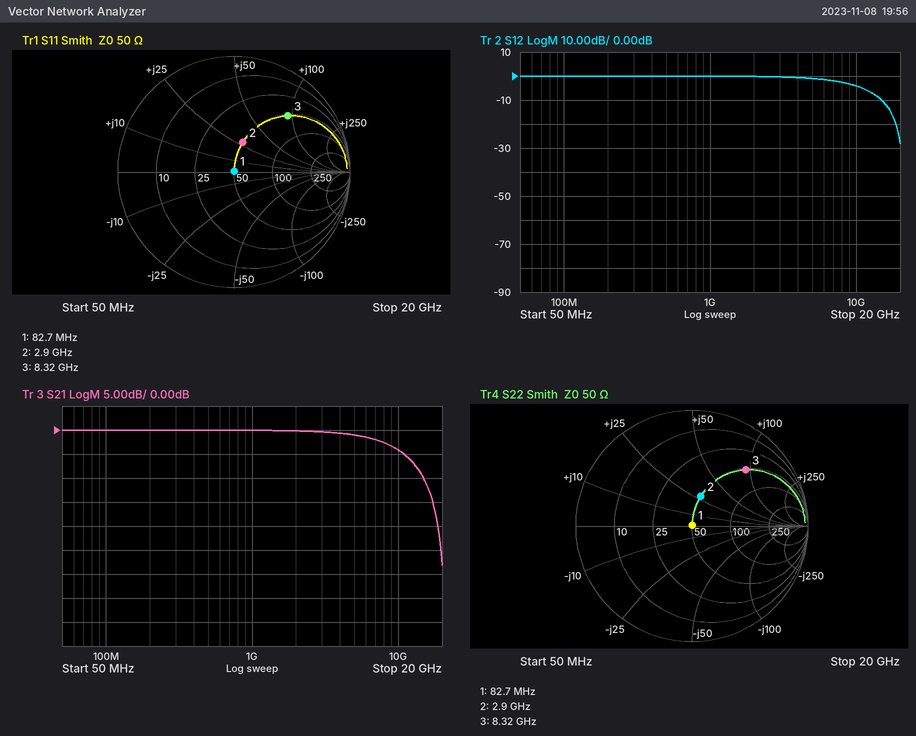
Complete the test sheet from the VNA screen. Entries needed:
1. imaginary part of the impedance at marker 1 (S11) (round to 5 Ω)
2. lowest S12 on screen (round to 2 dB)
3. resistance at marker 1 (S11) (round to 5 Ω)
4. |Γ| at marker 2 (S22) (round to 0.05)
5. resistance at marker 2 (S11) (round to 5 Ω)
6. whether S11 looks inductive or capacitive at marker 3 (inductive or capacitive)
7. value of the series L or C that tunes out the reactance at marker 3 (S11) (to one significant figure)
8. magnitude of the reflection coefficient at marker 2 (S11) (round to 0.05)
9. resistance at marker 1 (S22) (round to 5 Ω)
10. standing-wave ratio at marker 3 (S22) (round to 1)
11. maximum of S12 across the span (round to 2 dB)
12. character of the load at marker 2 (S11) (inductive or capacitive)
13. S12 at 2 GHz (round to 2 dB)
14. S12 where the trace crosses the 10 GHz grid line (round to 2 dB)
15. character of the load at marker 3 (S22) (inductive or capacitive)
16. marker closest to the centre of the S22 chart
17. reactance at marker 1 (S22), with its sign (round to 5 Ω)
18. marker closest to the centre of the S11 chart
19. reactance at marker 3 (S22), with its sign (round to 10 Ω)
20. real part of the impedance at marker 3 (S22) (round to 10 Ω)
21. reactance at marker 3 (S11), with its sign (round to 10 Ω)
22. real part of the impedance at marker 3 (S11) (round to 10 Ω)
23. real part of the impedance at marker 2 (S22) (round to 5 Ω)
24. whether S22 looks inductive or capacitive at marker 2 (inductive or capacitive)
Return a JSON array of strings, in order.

["0 Ω", "-28 dB", "50 Ω", "0.25", "50 Ω", "inductive", "200 fF", "0.25", "50 Ω", "5", "0 dB", "inductive", "0 dB", "-4 dB", "inductive", "marker 1", "0 Ω", "marker 1", "+90 Ω", "50 Ω", "+90 Ω", "50 Ω", "50 Ω", "inductive"]
